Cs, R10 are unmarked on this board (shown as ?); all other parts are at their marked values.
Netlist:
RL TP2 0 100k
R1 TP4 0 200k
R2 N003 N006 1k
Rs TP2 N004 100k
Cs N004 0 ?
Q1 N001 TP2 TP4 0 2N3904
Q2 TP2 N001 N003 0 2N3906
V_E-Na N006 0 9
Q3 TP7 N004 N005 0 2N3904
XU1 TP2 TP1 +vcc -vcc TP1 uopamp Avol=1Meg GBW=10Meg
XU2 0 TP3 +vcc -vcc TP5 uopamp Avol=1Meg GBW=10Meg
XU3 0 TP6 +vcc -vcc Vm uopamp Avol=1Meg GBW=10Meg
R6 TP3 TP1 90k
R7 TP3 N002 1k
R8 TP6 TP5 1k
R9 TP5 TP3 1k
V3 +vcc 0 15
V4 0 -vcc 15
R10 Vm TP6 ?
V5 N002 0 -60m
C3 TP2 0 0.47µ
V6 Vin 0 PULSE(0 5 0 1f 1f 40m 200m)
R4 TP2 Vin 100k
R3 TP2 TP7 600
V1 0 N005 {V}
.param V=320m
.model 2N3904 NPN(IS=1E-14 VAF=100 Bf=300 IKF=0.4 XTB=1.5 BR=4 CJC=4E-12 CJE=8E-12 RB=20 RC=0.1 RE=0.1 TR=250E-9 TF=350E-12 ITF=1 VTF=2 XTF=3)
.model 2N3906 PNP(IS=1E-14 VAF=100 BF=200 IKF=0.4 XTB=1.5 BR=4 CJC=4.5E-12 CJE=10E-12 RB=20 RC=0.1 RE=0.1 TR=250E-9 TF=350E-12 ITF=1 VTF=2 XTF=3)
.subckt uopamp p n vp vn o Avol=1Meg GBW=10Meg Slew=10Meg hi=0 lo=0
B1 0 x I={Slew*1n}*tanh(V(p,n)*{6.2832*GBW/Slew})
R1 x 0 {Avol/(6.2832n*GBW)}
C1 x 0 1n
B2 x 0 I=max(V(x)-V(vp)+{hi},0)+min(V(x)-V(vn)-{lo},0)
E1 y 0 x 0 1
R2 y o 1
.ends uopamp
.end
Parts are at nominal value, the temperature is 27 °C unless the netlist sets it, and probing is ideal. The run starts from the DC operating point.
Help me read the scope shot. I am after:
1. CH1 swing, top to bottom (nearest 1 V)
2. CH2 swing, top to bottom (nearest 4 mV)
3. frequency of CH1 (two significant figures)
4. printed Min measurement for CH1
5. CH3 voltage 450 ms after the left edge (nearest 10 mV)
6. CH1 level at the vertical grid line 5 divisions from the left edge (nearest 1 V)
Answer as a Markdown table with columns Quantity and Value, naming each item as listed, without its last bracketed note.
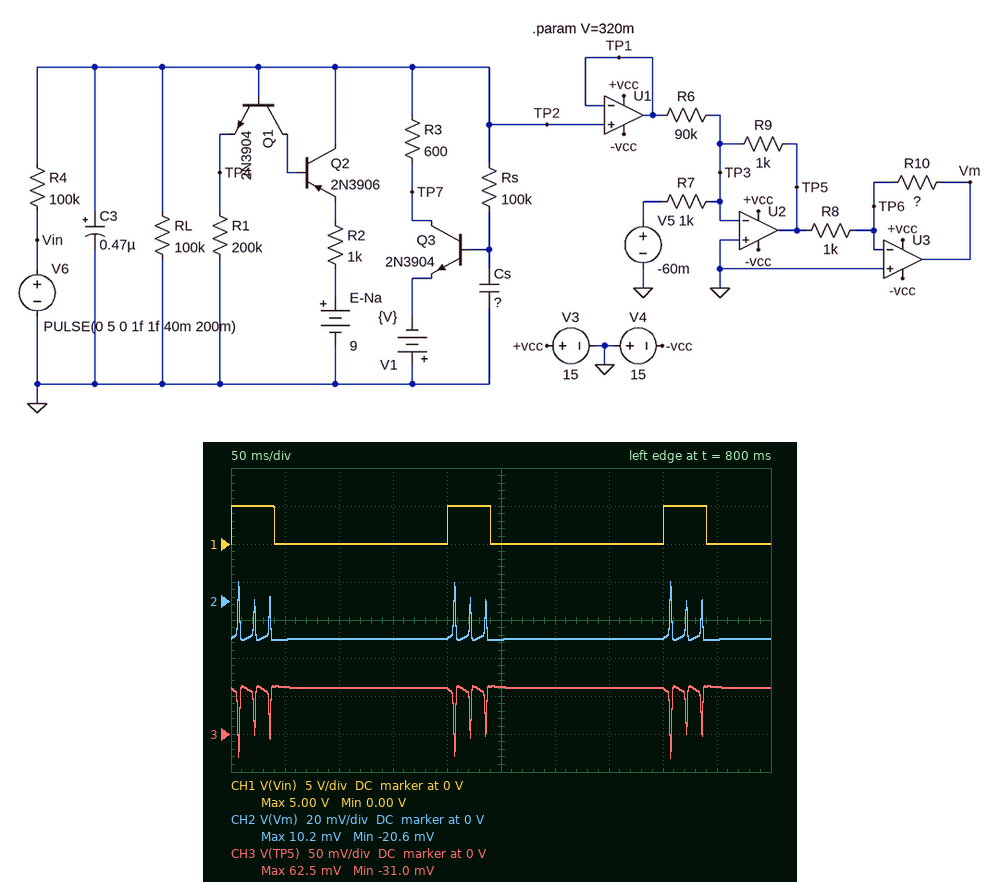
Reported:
| Quantity | Value |
|---|---|
| CH1 swing, top to bottom | 5 V |
| CH2 swing, top to bottom | 32 mV |
| frequency of CH1 | 5.0 Hz |
| printed Min measurement for CH1 | 0.00 V |
| CH3 voltage 450 ms after the left edge | 60 mV |
| CH1 level at the vertical grid line 5 divisions from the left edge | 0 V |
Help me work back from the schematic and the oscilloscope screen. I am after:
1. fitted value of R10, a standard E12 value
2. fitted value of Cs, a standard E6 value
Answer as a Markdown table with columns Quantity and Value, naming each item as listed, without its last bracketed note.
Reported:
| Quantity | Value |
|---|---|
| fitted value of R10, a standard E12 value | 330 Ω |
| fitted value of Cs, a standard E6 value | 330 nF |
